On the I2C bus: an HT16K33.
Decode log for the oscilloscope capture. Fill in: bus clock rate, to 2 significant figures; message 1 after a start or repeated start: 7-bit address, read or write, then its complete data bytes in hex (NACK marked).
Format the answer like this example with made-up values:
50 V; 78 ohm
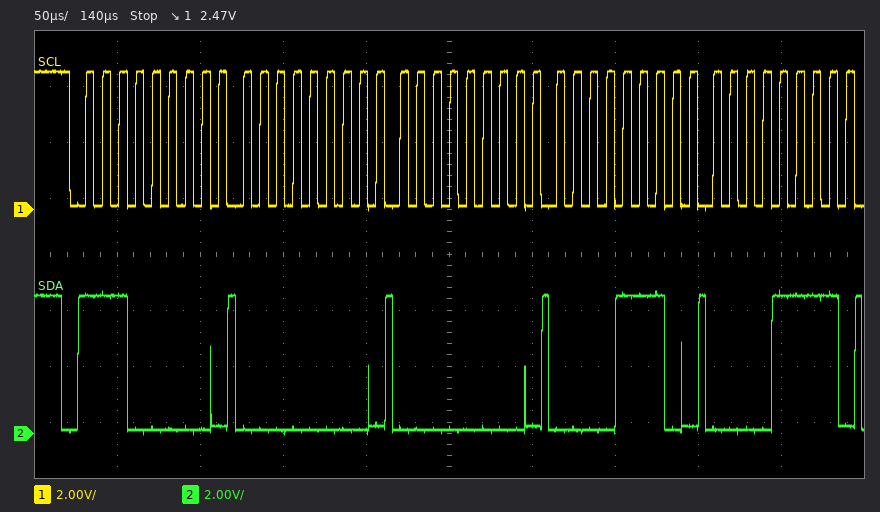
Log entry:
100 kHz; 0x70 write: 00 00 0E 0F
